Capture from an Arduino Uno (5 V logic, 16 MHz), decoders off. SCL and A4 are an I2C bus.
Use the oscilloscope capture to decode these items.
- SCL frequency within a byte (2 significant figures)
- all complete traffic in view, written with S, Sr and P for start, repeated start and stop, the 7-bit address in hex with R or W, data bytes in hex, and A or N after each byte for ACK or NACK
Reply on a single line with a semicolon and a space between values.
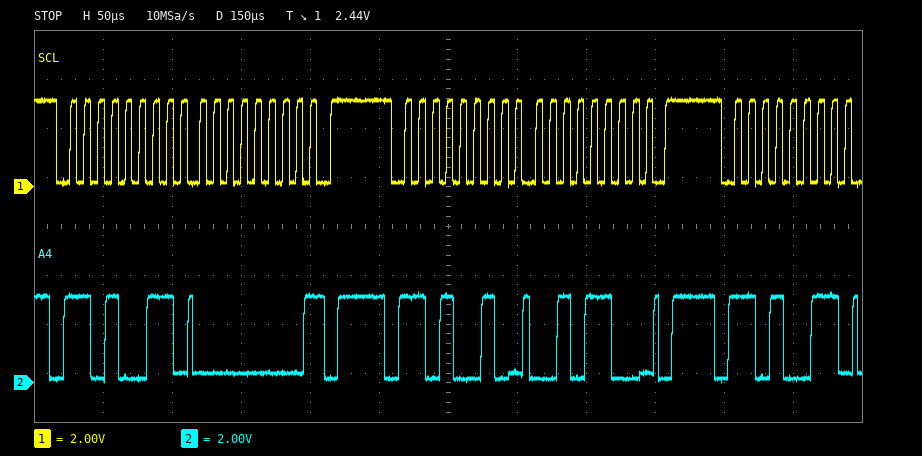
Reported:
100 kHz; S 69R A 00 N P S 69W A 2C A P S 69R A
